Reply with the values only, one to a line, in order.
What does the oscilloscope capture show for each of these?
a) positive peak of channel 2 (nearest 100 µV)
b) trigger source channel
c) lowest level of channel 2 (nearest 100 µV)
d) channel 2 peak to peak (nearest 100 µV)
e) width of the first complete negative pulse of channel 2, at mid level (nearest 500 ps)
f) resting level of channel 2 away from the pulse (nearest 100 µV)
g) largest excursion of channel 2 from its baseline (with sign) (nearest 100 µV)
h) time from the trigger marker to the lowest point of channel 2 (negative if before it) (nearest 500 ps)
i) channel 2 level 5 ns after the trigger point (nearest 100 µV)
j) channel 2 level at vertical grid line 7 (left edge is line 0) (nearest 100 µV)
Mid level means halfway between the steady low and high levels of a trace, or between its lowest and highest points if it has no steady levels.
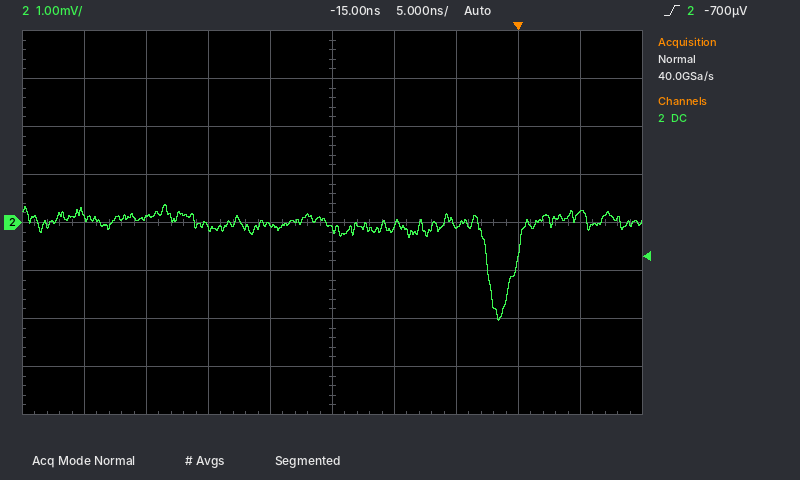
400 µV
channel 2
-2.0 mV
2.4 mV
2.5 ns
0.0 mV
-2.0 mV
-1.5 ns
200 µV
-100 µV
